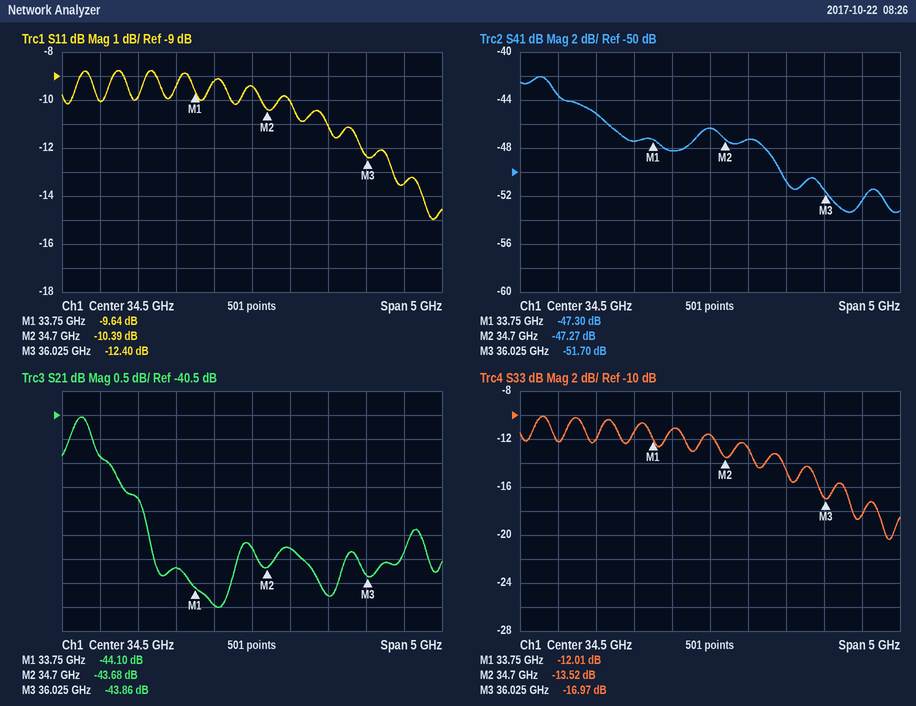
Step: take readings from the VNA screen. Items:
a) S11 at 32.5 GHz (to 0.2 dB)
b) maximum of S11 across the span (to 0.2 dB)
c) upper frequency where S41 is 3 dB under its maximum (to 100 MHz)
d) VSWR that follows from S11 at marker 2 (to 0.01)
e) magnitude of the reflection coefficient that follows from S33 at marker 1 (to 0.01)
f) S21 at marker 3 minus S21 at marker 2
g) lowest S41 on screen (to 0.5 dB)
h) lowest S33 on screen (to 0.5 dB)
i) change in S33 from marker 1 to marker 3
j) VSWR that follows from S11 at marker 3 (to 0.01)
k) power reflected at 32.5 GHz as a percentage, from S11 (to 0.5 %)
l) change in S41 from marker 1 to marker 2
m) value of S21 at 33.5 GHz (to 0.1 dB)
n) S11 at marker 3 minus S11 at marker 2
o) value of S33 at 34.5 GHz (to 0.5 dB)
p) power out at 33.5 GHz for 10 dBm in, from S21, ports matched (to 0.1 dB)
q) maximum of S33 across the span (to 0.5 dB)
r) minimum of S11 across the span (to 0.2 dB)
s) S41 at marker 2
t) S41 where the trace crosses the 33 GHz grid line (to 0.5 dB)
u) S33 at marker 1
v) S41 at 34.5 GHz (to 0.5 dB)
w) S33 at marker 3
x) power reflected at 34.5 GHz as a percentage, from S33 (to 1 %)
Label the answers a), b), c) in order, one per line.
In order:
a) -10.0 dB
b) -8.8 dB
c) 33.0 GHz
d) 1.87
e) 0.25
f) -0.18 dB
g) -53.5 dB
h) -20.5 dB
i) -4.96 dB
j) 1.63
k) 10.0 %
l) 0.03 dB
m) -43.7 dB
n) -2.01 dB
o) -11.5 dB
p) -33.7 dBm
q) -10.0 dB
r) -15.0 dB
s) -47.27 dB
t) -45.0 dB
u) -12.01 dB
v) -46.5 dB
w) -16.97 dB
x) 7 %
